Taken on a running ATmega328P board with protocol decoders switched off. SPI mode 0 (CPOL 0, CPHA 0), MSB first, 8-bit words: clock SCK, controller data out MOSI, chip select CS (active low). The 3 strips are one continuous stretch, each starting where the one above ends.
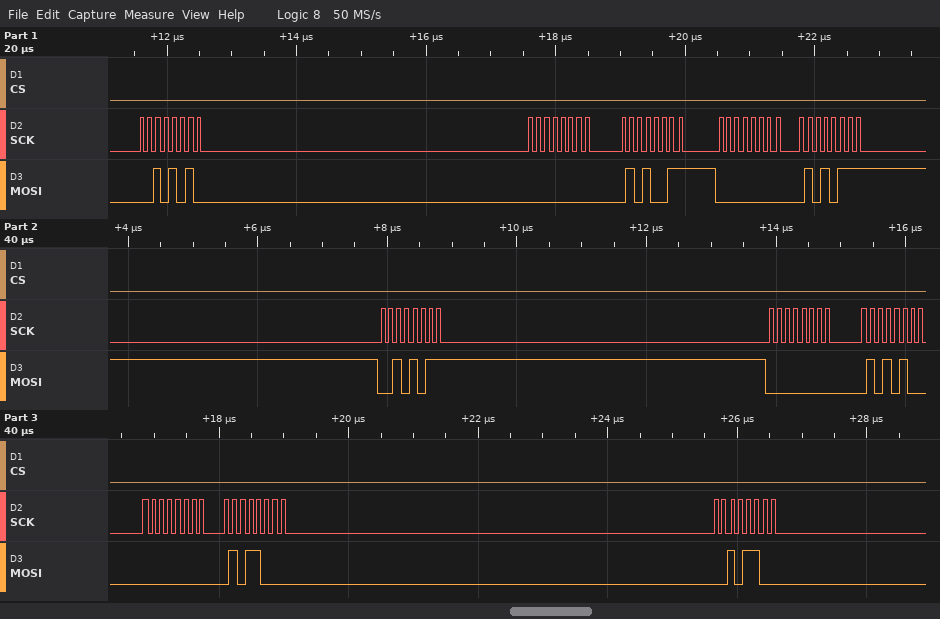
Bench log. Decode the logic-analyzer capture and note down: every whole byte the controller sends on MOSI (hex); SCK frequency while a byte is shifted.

0x2A 0x00 0x53 0x00 0x57 0x2B 0x00 0x54 0x00 0x58 0x2C
8 MHz
